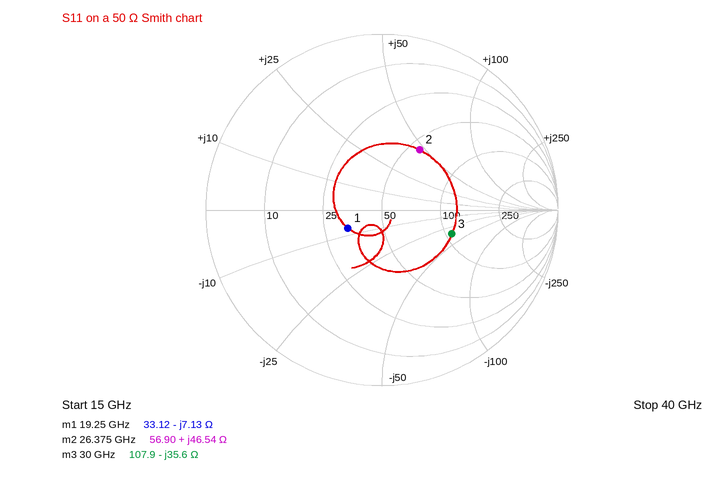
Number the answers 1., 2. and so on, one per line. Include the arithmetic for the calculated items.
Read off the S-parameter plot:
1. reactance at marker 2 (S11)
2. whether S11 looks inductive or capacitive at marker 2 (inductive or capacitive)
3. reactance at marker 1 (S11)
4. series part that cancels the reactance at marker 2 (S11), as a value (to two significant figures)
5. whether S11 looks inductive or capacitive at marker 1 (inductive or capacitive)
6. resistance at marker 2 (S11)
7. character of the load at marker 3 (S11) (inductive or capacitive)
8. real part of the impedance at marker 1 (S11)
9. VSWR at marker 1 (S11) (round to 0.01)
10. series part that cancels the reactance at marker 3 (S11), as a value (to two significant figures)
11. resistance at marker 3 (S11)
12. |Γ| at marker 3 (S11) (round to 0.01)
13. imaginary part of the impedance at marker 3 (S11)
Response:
1. +46.54 Ω
2. inductive
3. -7.13 Ω
4. C = 1/(2π × 26.375 GHz × 46.54 Ω) ≈ 130 fF
5. capacitive
6. 56.90 Ω
7. capacitive
8. 33.12 Ω
9. 1.56
10. L = 35.6 Ω/(2π × 30 GHz) ≈ 189 pH, so 190 pH to two significant figures
11. 107.9 Ω
12. 0.42
13. -35.6 Ω
